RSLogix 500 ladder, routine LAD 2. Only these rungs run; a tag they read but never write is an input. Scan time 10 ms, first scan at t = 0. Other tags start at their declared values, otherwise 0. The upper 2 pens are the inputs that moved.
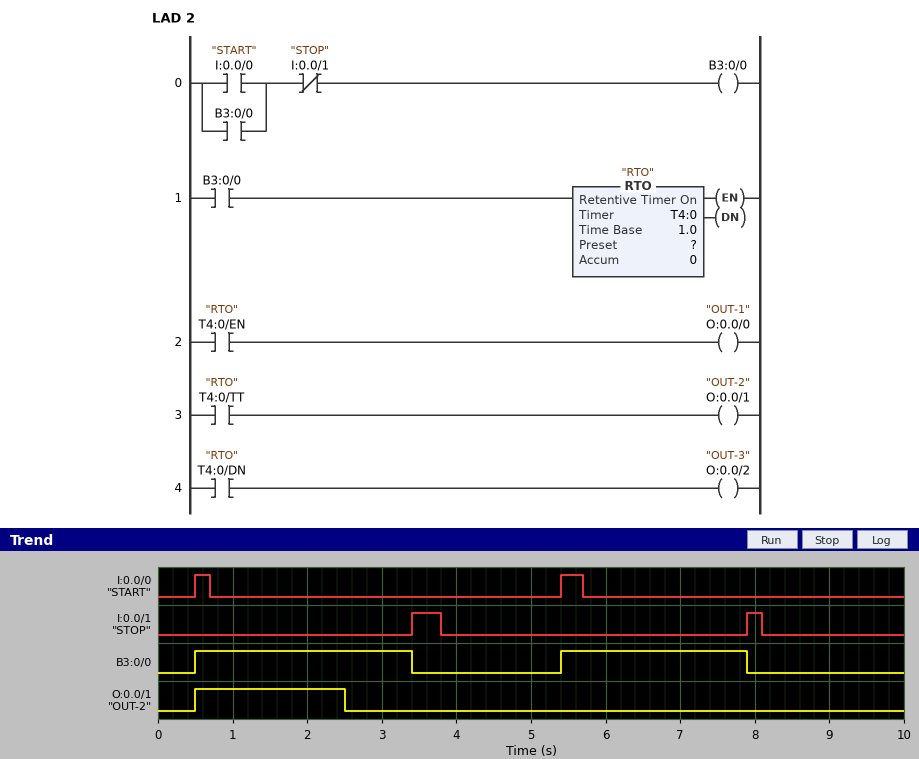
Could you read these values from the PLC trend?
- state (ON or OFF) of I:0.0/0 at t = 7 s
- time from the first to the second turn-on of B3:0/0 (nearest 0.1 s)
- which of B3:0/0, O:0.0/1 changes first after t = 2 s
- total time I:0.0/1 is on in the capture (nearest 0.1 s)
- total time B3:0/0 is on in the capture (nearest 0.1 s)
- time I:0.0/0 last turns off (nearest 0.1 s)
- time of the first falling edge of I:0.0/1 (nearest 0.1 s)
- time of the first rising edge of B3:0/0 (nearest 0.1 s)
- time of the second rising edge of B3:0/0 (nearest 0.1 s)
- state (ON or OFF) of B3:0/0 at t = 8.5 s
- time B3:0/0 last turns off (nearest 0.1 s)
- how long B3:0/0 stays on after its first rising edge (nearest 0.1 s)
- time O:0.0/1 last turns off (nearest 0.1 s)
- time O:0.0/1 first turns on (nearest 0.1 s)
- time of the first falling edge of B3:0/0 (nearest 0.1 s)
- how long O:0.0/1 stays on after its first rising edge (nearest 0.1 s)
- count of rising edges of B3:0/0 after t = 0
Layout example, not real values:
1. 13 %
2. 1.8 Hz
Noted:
1. OFF
2. 4.9 s
3. O:0.0/1
4. 0.6 s
5. 5.4 s
6. 5.7 s
7. 3.8 s
8. 0.5 s
9. 5.4 s
10. OFF
11. 7.9 s
12. 2.9 s
13. 2.5 s
14. 0.5 s
15. 3.4 s
16. 2.0 s
17. 2
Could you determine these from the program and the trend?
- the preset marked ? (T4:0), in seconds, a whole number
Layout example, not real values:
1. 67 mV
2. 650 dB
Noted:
1. 2 s
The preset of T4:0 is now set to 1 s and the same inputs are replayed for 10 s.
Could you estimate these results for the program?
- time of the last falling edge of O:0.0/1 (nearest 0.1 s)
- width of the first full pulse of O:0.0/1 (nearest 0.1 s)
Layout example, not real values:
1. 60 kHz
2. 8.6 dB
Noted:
1. 1.5 s
2. 1.0 s
